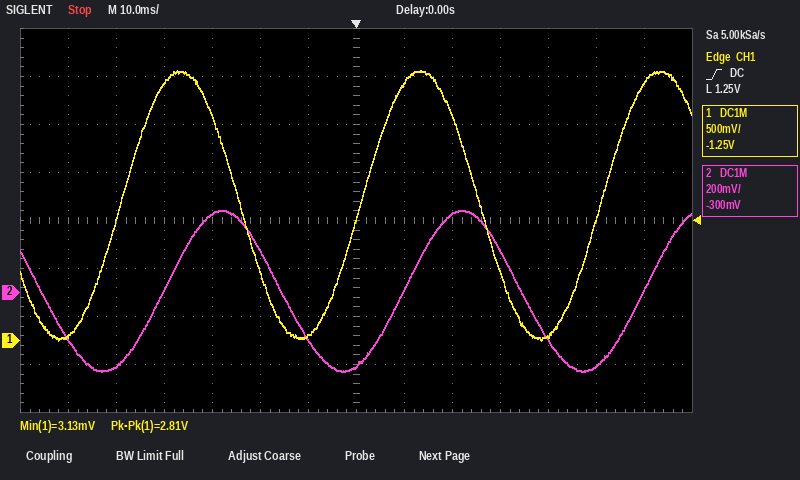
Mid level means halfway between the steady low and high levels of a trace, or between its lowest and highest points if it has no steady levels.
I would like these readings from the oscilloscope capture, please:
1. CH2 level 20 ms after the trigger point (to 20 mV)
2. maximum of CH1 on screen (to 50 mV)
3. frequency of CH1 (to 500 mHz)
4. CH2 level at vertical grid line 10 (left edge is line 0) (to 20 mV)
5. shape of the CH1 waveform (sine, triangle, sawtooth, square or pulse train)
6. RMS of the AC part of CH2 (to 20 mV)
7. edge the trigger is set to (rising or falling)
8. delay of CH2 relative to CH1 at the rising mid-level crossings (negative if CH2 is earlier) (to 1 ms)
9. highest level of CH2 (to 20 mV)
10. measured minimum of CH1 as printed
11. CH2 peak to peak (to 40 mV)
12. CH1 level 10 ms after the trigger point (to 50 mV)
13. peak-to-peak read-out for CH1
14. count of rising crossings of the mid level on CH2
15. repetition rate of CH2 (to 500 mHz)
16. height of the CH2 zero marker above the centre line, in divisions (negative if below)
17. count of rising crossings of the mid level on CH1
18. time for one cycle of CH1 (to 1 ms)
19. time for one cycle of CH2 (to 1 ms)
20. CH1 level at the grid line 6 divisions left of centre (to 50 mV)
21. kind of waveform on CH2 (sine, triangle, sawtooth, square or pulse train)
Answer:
320 mV
2.80 V
20.0 Hz
180 mV
sine
240 mV
rising
+9 ms
340 mV
3.13 mV
680 mV
2.70 V
2.81 V
3
20.0 Hz
-1.5 div
3
50 ms
50 ms
50 mV
sine
